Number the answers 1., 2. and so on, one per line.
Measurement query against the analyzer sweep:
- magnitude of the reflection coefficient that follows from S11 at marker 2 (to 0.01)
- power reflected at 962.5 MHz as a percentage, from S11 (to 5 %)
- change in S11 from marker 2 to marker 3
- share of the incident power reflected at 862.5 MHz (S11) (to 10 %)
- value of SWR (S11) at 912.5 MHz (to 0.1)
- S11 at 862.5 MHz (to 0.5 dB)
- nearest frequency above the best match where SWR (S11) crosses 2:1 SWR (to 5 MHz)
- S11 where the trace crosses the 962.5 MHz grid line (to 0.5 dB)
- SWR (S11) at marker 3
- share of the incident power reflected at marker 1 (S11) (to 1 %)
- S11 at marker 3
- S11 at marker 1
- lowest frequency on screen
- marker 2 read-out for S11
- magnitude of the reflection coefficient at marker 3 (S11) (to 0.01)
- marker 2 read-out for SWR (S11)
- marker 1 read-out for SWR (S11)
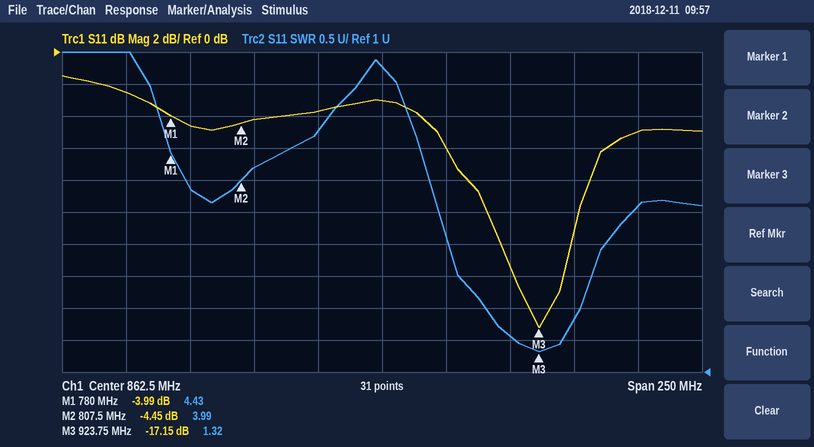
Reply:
1. 0.60
2. 30 %
3. -12.70 dB
4. 50 %
5. 1.6
6. -3.0 dB
7. 940 MHz
8. -5.0 dB
9. 1.32
10. 40 %
11. -17.15 dB
12. -3.99 dB
13. 737.5 MHz
14. -4.45 dB
15. 0.14
16. 3.99
17. 4.43
